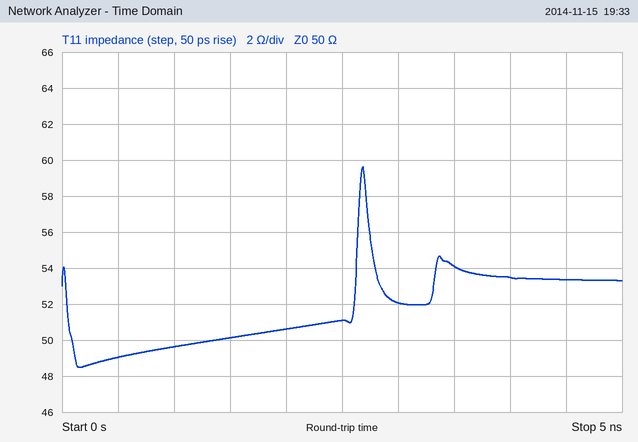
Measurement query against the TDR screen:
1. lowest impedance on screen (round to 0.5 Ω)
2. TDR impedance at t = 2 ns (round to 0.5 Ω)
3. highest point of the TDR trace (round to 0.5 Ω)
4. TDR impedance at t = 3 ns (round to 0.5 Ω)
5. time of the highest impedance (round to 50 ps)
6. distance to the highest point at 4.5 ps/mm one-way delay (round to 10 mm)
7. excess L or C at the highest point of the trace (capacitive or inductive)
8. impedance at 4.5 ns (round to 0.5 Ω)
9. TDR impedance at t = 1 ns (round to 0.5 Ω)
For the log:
48.5 Ω
50.5 Ω
59.5 Ω
52.0 Ω
2.70 ns
300 mm
inductive
53.5 Ω
49.5 Ω
